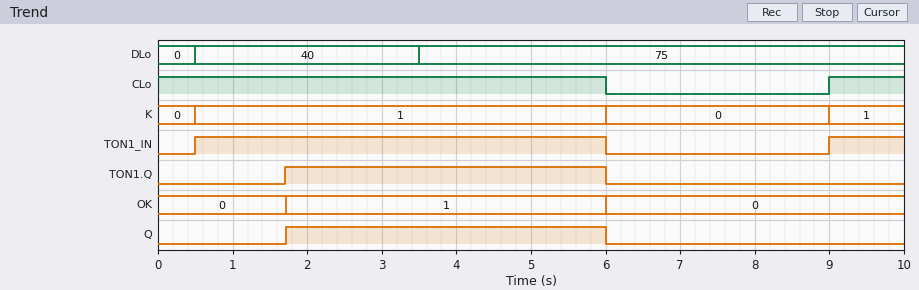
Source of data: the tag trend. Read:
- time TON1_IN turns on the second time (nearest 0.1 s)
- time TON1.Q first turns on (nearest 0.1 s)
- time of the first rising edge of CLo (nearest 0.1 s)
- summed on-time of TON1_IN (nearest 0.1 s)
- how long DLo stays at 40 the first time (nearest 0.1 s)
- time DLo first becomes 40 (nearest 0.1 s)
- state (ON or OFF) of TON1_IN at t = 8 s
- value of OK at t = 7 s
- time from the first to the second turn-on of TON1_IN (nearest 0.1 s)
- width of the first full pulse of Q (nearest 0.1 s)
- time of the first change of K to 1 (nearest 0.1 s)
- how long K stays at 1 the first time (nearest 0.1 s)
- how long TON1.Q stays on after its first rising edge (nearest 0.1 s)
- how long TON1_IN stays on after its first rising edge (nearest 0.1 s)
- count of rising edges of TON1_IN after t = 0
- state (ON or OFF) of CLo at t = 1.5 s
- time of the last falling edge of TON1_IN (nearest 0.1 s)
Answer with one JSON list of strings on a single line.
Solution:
["9.0 s", "1.7 s", "9.0 s", "6.5 s", "3.0 s", "0.5 s", "OFF", "0", "8.5 s", "4.3 s", "0.5 s", "5.5 s", "4.3 s", "5.5 s", "2", "ON", "6.0 s"]
